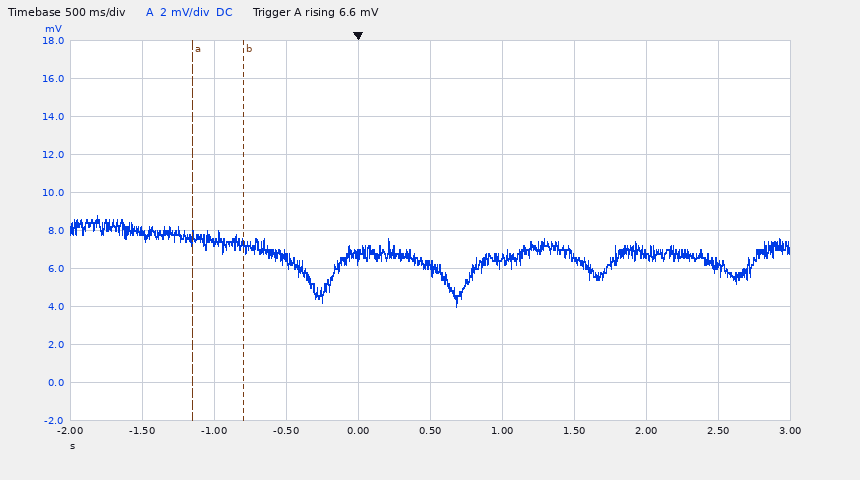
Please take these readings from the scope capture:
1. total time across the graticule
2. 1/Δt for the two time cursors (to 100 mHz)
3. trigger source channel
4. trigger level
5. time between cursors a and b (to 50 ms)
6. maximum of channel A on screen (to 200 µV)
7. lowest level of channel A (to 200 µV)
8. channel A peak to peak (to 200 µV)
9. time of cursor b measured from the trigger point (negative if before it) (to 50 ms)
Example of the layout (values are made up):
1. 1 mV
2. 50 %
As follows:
1. 5 s
2. 2.9 Hz
3. channel A
4. 6.6 mV
5. 350 ms
6. 8.8 mV
7. 4.0 mV
8. 4.8 mV
9. -800 ms
